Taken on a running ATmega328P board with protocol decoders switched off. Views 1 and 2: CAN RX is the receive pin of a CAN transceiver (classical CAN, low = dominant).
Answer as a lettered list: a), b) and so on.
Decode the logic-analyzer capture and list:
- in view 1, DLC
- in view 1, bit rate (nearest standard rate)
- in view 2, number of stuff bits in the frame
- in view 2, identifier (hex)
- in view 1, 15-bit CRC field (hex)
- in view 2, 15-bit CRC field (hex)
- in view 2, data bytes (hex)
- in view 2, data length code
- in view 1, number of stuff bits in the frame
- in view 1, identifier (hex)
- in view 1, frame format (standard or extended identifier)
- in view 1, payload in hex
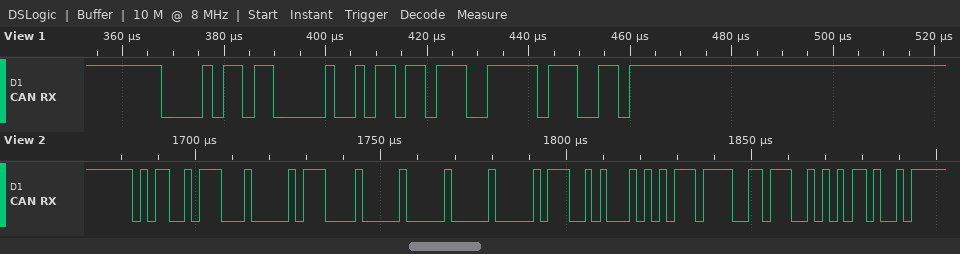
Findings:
a) 1
b) 500 kbit/s
c) 5
d) 0x597
e) 0x67F9
f) 0x4AB4
g) 1C 20 00 00 E5 15 77 9B
h) 8
i) 2
j) 0x0B6
k) standard
l) 6D
